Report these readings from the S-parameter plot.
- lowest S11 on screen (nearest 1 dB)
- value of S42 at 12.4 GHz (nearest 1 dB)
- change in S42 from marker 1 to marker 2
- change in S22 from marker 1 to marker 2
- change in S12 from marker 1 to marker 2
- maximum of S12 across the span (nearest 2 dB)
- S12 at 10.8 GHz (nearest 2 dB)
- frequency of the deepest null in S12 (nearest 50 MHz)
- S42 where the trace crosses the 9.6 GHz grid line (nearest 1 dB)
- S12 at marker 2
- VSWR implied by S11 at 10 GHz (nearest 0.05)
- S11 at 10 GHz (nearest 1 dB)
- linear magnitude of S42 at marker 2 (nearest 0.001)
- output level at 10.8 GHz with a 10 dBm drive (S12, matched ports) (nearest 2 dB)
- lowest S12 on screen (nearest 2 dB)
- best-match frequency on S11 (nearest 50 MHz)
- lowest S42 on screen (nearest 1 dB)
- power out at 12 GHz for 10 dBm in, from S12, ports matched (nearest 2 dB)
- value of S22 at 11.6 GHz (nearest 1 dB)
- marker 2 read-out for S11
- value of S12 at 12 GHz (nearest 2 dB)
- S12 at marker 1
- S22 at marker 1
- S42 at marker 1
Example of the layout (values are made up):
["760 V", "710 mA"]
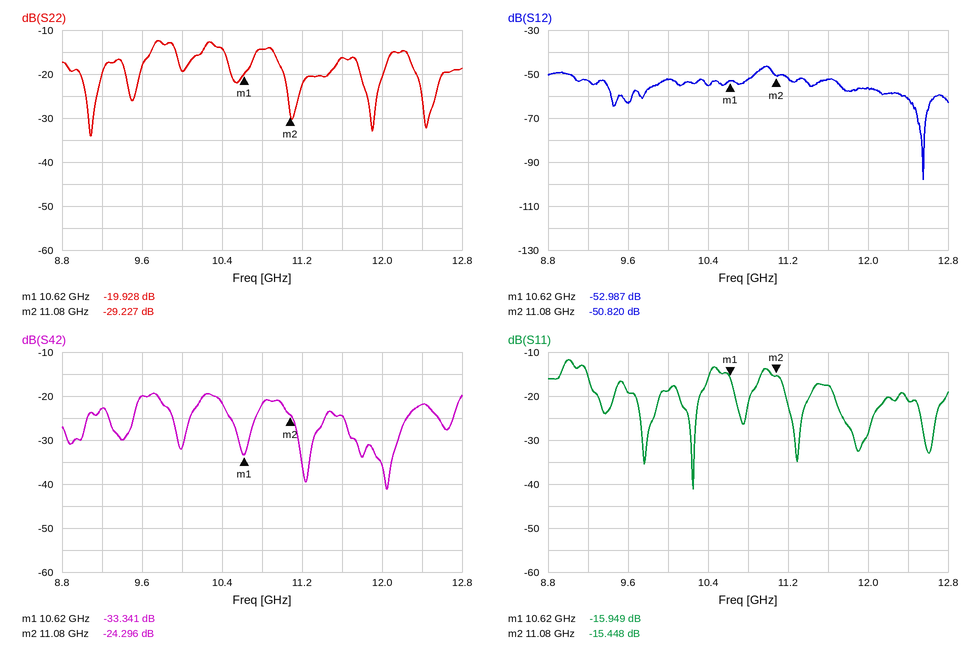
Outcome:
["-41 dB", "-22 dB", "9.045 dB", "-9.299 dB", "2.167 dB", "-46 dB", "-52 dB", "12.55 GHz", "-20 dB", "-50.820 dB", "1.25", "-19 dB", "0.061", "-42 dBm", "-98 dB", "10.25 GHz", "-41 dB", "-46 dBm", "-16 dB", "-15.448 dB", "-56 dB", "-52.987 dB", "-19.928 dB", "-33.341 dB"]
